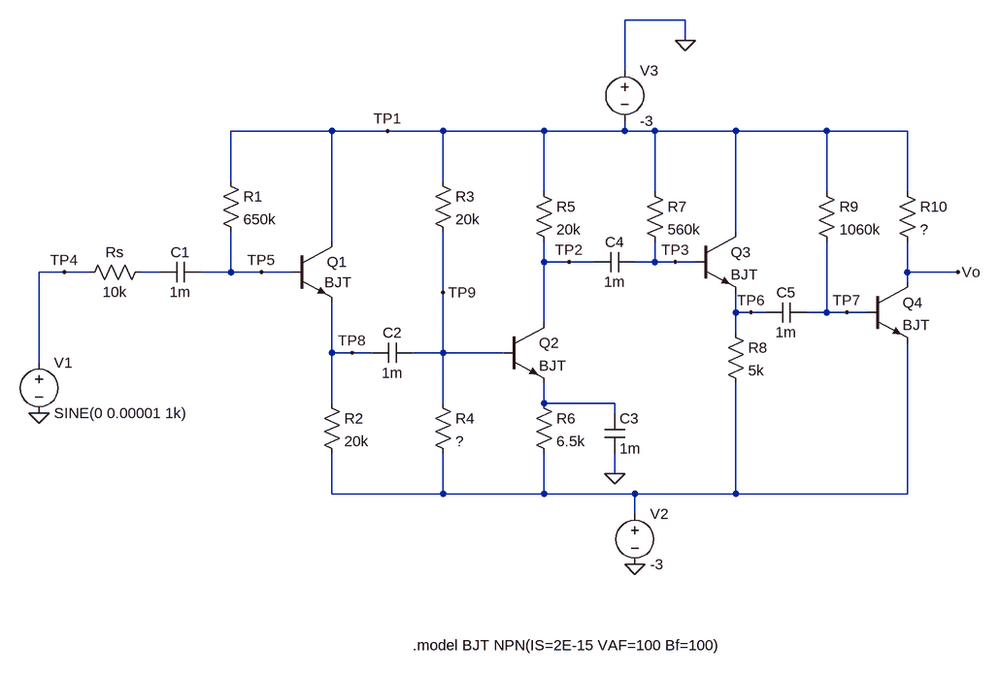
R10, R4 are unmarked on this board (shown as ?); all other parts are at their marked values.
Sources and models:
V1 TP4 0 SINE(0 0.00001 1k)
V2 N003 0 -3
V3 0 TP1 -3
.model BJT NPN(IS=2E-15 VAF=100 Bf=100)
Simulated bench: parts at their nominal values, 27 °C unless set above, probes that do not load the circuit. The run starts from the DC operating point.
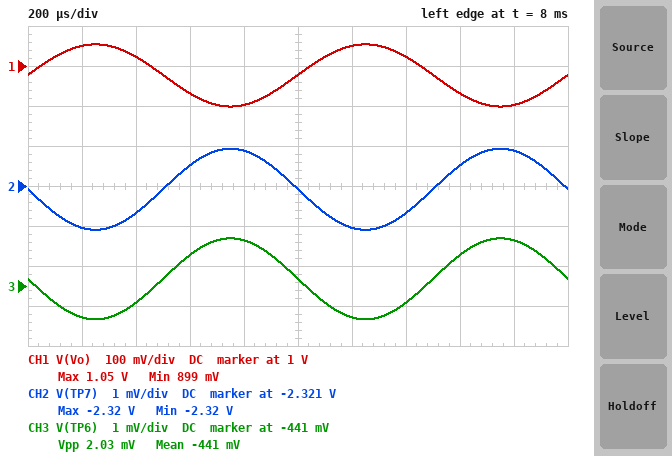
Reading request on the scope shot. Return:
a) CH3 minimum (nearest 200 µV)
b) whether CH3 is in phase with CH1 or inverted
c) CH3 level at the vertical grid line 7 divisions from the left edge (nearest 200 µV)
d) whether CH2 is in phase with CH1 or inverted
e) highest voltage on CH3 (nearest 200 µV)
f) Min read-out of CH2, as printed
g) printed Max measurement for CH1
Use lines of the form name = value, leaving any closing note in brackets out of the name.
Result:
CH3 minimum = -441.8 mV
whether CH3 is in phase with CH1 or inverted = inverted
CH3 level at the vertical grid line 7 divisions from the left edge = -441.4 mV
whether CH2 is in phase with CH1 or inverted = inverted
highest voltage on CH3 = -439.8 mV
Min read-out of CH2, as printed = -2.32 V
printed Max measurement for CH1 = 1.05 V
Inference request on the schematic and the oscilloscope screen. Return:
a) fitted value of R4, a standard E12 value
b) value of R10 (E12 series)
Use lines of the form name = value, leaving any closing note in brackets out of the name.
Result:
fitted value of R4, a standard E12 value = 8.2 kΩ
value of R10 = 3.9 kΩ
